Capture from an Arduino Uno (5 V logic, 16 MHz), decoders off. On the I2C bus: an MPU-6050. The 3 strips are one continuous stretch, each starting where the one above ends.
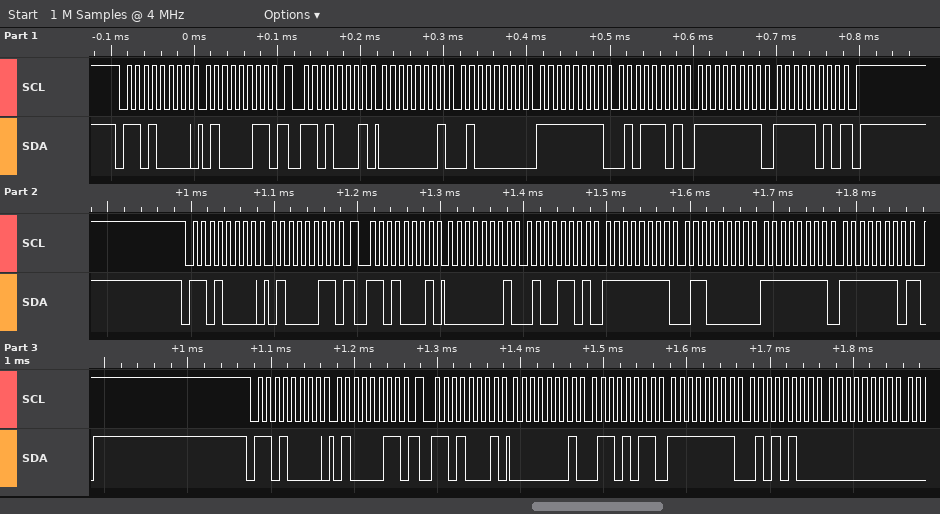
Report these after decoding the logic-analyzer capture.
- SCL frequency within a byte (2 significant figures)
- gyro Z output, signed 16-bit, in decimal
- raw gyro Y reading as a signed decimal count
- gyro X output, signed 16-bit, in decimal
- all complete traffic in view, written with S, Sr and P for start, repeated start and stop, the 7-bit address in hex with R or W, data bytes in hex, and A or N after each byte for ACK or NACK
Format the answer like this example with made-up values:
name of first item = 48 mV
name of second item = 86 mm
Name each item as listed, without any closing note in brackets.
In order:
SCL frequency within a byte = 100 kHz
gyro Z output, signed 16-bit, in decimal = -6
raw gyro Y reading as a signed decimal count = -163
gyro X output, signed 16-bit, in decimal = 320
all complete traffic in view, written with S, Sr and P for start, repeated start and stop, the 7-bit address in hex with R or W, data bytes in hex, and A or N after each byte for ACK or NACK = S 68W A 43 A Sr 68R A 01 A 40 A FF A 5D A FF A FA N P S 68W A 43 A Sr 68R A 01 A 4D A FF A 60 A FF A FE N P S 68W A 43 A Sr 68R A 01 A 6B A FF A 54 A 00 A
